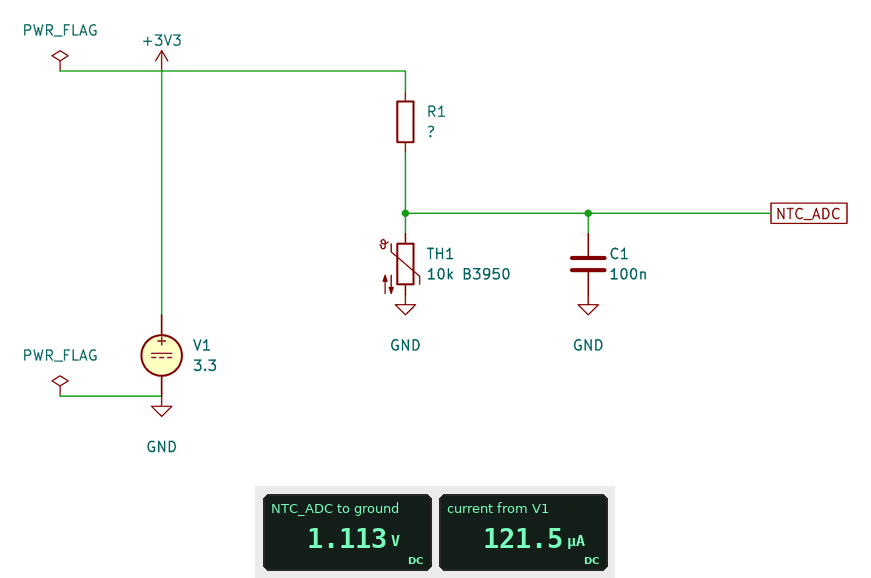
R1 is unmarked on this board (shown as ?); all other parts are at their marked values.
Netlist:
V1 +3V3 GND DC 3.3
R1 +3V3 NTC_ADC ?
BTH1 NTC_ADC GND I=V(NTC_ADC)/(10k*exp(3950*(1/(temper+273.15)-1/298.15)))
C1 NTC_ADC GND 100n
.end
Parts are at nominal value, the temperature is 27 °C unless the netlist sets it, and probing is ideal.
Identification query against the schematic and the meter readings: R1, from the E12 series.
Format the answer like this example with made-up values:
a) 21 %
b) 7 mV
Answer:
a) 18 kΩ
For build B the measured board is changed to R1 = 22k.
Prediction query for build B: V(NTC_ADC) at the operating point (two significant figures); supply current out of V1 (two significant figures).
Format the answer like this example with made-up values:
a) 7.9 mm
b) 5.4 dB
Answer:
a) 970 mV
b) 110 µA
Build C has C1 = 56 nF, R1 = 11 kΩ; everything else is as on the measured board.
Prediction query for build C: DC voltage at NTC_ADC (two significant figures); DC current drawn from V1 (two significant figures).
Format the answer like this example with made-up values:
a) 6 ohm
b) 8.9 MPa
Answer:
a) 1.5 V
b) 160 µA
